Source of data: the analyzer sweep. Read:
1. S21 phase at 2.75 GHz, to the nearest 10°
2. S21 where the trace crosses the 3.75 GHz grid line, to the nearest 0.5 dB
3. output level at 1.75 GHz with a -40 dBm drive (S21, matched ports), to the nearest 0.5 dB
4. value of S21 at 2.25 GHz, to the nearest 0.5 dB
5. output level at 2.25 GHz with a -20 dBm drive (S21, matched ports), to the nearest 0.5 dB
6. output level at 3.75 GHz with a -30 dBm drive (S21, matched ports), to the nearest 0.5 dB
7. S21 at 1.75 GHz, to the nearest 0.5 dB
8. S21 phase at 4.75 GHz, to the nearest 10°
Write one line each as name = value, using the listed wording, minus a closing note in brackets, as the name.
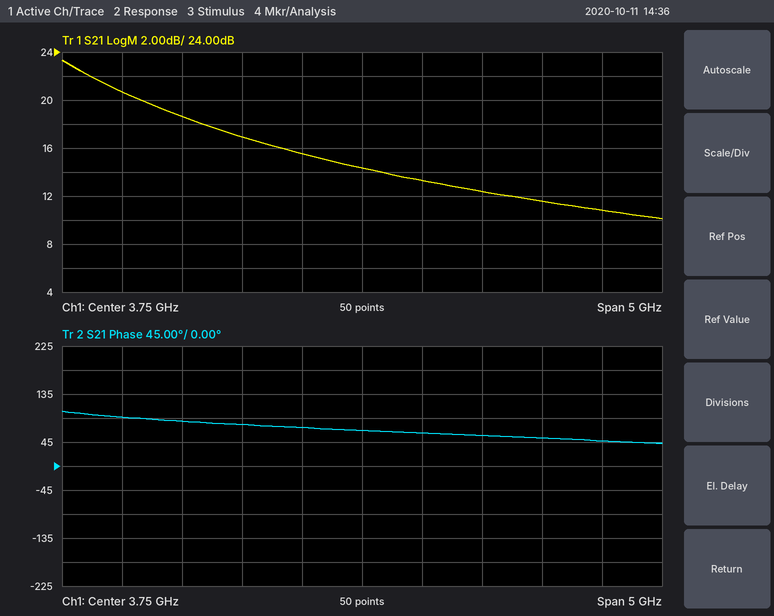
S21 phase at 2.75 GHz, to the nearest 10° = 80°
S21 where the trace crosses the 3.75 GHz grid line, to the nearest 0.5 dB = 14.5 dB
output level at 1.75 GHz with a -40 dBm drive (S21, matched ports), to the nearest 0.5 dB = -19.5 dBm
value of S21 at 2.25 GHz, to the nearest 0.5 dB = 18.5 dB
output level at 2.25 GHz with a -20 dBm drive (S21, matched ports), to the nearest 0.5 dB = -1.5 dBm
output level at 3.75 GHz with a -30 dBm drive (S21, matched ports), to the nearest 0.5 dB = -15.5 dBm
S21 at 1.75 GHz, to the nearest 0.5 dB = 20.5 dB
S21 phase at 4.75 GHz, to the nearest 10° = 60°
